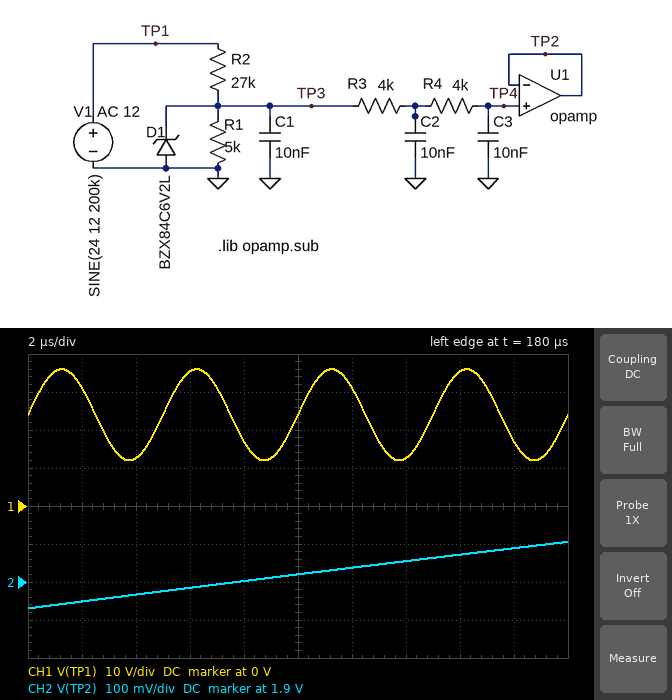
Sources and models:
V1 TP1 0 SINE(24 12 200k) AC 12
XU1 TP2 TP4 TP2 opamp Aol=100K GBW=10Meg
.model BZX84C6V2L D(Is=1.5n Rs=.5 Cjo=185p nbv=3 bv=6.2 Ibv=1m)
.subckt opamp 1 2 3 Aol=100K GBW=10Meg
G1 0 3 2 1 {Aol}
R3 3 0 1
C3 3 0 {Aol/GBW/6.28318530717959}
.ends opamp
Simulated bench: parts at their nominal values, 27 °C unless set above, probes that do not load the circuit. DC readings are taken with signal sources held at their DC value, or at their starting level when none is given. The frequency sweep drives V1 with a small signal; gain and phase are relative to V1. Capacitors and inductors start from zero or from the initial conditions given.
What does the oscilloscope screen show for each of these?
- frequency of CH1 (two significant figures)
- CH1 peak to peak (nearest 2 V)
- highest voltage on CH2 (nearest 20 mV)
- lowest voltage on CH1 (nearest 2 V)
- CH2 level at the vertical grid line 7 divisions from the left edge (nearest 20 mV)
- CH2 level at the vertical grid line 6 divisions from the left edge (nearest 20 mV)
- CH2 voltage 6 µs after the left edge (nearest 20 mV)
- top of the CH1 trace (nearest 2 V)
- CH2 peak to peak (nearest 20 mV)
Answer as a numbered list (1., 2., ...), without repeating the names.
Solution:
1. 200 kHz
2. 24 V
3. 2.00 V
4. 12 V
5. 1.96 V
6. 1.94 V
7. 1.88 V
8. 36 V
9. 180 mV
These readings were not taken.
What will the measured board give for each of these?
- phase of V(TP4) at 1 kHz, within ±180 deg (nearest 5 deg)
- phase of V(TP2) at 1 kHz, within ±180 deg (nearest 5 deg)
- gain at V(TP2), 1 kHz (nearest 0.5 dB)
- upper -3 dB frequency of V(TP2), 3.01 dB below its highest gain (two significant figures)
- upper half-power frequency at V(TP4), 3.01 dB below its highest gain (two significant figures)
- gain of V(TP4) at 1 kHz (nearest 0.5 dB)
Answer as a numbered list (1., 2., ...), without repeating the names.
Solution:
1. -65 deg
2. -65 deg
3. -20.5 dB
4. 750 Hz
5. 750 Hz
6. -20.5 dB
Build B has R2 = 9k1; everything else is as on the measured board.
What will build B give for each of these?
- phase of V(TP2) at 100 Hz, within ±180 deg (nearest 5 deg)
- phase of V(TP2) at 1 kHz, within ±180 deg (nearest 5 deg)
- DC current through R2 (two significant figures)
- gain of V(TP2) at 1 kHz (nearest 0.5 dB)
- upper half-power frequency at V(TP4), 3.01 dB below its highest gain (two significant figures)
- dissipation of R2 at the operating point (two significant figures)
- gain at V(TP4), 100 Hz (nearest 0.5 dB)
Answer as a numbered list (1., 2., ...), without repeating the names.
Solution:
1. -5 deg
2. -40 deg
3. 2.0 mA
4. -40.5 dB
5. 1.5 kHz
6. 35 mW
7. -39.0 dB
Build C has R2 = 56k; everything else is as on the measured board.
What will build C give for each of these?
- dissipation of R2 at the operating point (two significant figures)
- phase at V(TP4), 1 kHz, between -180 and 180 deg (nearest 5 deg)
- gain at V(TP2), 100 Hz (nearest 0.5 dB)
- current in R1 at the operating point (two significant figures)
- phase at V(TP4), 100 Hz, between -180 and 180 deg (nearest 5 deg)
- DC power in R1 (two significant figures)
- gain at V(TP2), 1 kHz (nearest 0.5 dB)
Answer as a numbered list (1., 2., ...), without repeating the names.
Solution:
1. 8.7 mW
2. -70 deg
3. -22.0 dB
4. 390 µA
5. -10 deg
6. 770 µW
7. -26.5 dB
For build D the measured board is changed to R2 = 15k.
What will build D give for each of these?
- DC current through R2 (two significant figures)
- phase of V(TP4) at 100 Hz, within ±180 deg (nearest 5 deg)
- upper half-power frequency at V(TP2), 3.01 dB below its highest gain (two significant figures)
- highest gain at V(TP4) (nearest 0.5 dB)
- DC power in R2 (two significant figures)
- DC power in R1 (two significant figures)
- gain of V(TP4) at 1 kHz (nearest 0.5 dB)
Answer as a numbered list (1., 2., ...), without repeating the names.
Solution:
1. 1.2 mA
2. -5 deg
3. 1.1 kHz
4. -18.5 dB
5. 22 mW
6. 7.0 mW
7. -21.5 dB
